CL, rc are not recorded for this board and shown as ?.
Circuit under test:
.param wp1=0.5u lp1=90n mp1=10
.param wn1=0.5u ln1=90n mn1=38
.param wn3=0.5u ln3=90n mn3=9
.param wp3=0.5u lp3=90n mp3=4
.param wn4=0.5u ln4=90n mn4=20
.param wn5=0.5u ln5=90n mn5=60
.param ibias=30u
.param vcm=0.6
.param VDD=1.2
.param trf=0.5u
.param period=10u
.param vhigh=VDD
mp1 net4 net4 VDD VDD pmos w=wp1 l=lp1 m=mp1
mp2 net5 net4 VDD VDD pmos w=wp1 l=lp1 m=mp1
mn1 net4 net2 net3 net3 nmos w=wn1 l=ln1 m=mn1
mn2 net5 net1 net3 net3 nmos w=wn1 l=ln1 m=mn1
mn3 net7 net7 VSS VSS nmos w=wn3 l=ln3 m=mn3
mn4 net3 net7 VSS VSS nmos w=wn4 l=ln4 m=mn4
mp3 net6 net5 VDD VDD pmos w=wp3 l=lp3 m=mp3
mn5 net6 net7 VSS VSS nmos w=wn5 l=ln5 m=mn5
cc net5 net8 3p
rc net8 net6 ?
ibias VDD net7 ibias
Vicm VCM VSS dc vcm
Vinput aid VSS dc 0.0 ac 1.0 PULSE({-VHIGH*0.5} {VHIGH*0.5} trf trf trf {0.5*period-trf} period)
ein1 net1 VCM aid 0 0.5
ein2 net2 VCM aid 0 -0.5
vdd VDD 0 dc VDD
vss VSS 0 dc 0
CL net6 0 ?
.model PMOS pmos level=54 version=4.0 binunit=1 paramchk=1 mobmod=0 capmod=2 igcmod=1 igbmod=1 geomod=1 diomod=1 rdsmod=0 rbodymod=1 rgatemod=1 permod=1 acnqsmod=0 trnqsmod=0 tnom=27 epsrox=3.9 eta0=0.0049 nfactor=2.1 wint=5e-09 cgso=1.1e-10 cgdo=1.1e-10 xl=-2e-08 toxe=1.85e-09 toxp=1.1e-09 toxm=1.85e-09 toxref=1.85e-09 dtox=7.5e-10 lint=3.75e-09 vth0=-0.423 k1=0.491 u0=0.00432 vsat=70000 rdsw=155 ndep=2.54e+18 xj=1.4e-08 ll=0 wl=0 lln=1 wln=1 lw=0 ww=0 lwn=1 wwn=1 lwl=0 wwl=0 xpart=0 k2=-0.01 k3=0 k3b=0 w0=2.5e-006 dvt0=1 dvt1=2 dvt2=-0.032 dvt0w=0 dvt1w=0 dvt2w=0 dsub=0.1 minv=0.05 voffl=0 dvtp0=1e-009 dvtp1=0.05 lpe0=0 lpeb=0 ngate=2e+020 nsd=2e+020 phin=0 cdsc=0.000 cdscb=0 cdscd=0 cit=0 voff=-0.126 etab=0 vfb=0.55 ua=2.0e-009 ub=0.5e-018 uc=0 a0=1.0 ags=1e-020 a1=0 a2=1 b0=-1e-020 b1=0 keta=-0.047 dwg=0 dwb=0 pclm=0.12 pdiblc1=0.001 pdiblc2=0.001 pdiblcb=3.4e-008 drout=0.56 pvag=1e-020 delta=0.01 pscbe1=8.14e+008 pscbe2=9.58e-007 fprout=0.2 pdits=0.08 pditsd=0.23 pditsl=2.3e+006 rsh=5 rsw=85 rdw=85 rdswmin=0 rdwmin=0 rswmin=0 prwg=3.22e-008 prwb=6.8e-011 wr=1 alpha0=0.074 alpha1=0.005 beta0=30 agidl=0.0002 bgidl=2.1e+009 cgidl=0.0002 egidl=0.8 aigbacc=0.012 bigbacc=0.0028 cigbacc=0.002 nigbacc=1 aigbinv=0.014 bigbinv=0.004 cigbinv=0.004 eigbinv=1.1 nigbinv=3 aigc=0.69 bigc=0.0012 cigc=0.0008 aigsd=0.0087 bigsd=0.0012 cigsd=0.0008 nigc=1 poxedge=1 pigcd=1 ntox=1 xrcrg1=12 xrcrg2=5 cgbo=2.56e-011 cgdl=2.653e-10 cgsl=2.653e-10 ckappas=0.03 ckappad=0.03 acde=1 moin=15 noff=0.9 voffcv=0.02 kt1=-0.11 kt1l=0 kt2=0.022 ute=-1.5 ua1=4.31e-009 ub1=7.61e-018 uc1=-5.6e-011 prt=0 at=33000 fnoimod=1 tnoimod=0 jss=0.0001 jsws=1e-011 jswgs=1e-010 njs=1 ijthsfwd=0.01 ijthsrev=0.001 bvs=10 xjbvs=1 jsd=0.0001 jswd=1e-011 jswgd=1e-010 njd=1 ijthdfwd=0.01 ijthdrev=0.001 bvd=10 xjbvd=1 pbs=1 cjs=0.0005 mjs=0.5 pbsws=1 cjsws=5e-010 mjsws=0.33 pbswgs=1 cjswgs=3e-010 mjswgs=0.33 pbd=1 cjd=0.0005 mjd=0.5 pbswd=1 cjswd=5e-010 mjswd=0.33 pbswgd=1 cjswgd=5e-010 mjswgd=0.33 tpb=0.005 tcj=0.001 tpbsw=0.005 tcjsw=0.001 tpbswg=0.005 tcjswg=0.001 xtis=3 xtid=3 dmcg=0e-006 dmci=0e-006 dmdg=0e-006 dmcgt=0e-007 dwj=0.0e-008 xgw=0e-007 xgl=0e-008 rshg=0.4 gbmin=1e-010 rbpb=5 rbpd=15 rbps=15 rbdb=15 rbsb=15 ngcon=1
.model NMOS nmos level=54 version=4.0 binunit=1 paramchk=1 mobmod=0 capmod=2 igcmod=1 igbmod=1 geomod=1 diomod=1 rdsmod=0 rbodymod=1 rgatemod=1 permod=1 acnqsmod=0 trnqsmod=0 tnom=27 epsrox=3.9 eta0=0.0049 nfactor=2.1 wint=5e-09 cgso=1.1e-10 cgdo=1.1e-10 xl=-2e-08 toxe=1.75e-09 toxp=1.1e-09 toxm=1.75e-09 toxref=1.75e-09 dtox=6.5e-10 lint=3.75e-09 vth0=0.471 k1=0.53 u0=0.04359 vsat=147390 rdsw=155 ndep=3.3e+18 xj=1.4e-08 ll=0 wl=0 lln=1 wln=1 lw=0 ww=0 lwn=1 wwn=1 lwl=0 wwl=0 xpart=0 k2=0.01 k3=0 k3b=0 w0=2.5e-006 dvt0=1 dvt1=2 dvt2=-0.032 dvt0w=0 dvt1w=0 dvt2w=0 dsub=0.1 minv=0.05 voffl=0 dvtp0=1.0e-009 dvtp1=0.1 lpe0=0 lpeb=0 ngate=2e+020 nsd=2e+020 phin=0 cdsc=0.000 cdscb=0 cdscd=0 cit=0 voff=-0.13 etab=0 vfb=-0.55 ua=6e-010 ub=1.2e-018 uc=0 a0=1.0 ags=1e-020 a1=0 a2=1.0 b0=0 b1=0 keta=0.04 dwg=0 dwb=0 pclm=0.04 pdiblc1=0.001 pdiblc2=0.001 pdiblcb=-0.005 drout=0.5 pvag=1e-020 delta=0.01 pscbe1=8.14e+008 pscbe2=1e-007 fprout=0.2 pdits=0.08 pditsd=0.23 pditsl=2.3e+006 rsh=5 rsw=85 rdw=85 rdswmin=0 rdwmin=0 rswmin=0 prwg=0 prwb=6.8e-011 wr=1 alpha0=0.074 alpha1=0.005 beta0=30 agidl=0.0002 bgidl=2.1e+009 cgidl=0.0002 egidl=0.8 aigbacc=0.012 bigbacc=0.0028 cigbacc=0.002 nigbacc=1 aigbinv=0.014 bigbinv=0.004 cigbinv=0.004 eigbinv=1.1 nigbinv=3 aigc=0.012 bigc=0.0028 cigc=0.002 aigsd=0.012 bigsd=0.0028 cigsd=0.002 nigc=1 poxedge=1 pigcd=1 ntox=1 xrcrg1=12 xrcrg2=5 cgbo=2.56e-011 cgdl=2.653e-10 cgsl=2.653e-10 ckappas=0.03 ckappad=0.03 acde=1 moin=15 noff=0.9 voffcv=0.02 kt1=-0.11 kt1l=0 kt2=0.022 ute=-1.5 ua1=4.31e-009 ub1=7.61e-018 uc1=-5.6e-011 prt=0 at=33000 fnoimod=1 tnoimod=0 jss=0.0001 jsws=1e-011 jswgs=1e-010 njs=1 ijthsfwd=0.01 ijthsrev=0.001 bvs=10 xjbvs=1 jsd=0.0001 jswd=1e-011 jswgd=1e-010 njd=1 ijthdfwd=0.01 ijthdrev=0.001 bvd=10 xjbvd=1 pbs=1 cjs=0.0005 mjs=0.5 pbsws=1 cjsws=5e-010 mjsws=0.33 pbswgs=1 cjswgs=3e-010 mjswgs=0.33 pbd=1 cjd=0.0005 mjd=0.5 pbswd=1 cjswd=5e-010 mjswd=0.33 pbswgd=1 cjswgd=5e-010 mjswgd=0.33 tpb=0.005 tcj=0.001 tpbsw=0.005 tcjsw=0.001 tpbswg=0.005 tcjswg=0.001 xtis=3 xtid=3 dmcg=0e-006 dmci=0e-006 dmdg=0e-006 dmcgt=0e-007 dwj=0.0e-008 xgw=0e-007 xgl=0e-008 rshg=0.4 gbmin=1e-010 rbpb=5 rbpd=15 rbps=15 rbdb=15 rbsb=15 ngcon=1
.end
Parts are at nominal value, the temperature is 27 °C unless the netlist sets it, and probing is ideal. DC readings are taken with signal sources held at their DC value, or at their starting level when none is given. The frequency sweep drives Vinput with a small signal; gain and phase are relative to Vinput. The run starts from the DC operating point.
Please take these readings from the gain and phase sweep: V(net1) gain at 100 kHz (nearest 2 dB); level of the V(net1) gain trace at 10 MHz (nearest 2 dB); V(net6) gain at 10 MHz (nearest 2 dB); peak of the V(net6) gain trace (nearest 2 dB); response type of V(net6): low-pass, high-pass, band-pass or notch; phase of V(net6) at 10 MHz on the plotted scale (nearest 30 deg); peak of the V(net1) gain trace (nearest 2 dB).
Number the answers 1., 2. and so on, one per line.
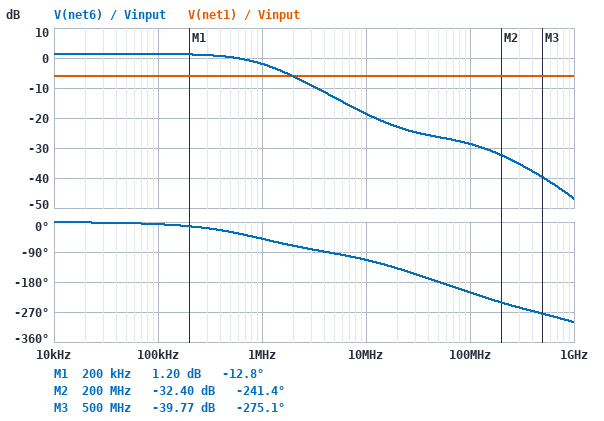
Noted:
1. -6 dB
2. -6 dB
3. -18 dB
4. 2 dB
5. low-pass
6. -120 deg
7. -6 dB
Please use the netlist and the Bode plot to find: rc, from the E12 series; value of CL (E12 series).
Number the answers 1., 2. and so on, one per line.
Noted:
1. 3.3 kΩ
2. 6.8 pF
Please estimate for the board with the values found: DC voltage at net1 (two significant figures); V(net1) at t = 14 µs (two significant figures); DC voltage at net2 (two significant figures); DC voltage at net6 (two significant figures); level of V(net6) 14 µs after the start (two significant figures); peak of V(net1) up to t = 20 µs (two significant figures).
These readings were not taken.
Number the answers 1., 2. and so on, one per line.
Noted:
1. 600 mV
2. 900 mV
3. 600 mV
4. 3.0 mV
5. 810 mV
6. 900 mV
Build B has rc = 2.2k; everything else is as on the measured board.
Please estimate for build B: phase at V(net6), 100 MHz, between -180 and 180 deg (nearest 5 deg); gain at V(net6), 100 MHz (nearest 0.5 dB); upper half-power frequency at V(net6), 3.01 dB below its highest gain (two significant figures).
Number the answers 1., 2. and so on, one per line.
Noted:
1. 145 deg
2. -25.0 dB
3. 950 kHz
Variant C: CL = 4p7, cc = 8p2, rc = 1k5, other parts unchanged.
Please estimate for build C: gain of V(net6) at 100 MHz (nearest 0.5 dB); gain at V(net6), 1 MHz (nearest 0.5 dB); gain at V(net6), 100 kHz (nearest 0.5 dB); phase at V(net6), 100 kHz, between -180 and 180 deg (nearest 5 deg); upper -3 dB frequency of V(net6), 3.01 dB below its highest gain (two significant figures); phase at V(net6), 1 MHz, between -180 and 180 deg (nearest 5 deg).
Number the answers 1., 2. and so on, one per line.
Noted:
1. -22.5 dB
2. -8.0 dB
3. 1.0 dB
4. -15 deg
5. 350 kHz
6. -85 deg
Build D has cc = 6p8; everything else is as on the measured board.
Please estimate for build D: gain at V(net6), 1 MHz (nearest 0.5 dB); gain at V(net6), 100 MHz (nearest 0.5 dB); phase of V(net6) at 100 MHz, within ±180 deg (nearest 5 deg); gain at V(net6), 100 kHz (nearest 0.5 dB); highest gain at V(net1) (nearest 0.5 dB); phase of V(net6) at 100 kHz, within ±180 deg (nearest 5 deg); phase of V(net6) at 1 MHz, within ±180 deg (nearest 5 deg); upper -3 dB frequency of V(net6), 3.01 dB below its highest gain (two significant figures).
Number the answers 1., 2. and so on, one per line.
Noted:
1. -7.0 dB
2. -29.0 dB
3. 140 deg
4. 1.0 dB
5. -6.0 dB
6. -15 deg
7. -75 deg
8. 410 kHz
